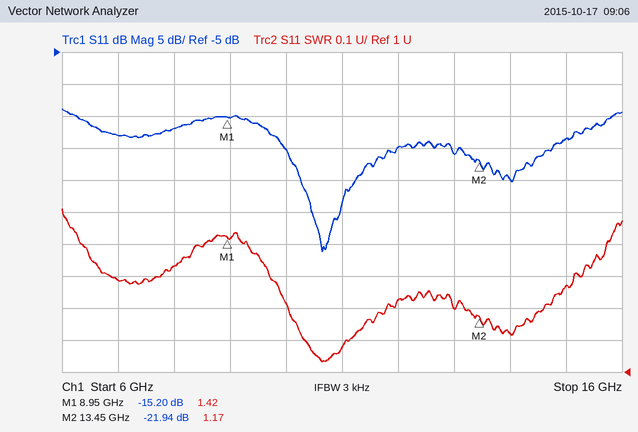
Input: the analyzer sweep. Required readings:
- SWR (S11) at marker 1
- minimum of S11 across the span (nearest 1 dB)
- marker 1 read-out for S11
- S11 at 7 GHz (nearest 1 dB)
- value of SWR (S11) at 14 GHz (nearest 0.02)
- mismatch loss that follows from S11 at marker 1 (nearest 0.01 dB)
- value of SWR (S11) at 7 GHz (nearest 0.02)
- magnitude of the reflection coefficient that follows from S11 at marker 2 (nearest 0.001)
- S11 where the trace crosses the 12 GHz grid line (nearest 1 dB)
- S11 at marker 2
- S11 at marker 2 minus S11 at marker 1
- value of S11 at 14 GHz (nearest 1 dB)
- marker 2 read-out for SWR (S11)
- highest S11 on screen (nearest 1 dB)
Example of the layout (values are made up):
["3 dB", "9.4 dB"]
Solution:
["1.42", "-36 dB", "-15.20 dB", "-18 dB", "1.12", "0.13 dB", "1.28", "0.080", "-20 dB", "-21.94 dB", "-6.74 dB", "-25 dB", "1.17", "-14 dB"]
